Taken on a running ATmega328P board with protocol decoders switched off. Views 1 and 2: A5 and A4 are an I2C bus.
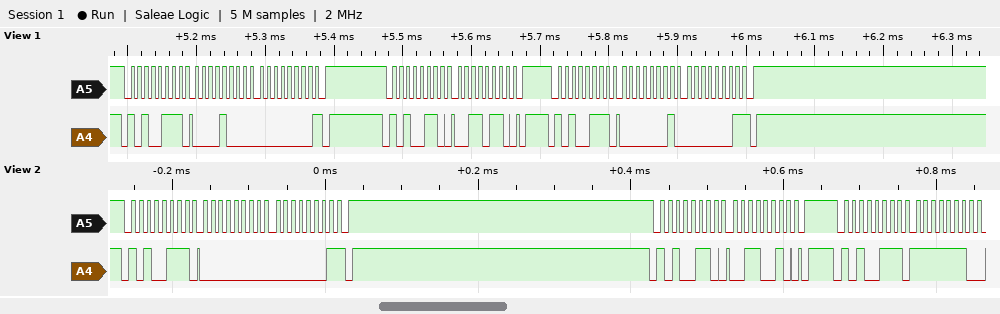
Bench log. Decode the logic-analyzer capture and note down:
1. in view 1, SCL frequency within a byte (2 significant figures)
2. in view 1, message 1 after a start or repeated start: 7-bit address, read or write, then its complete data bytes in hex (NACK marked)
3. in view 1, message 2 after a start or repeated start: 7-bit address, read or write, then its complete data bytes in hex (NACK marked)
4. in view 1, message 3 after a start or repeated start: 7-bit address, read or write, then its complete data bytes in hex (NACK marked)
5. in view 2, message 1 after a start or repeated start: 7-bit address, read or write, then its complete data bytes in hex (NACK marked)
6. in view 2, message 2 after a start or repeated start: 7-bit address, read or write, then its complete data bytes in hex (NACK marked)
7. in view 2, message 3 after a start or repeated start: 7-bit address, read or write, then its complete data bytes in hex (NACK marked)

100 kHz
0x53 read: 08 00 NACK
0x53 write: 36
0x53 read: 01 01 NACK
0x53 read: 00 01 NACK
0x53 write: 32
0x53 read: FE
